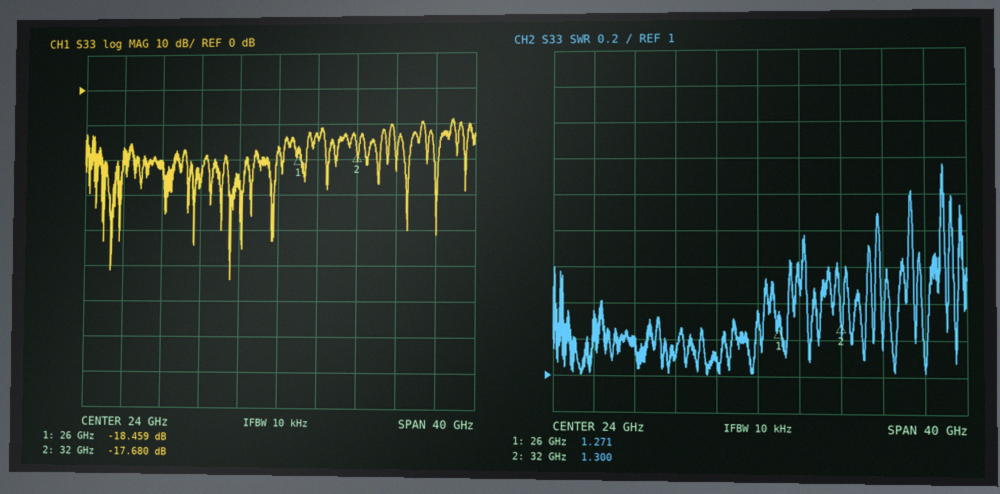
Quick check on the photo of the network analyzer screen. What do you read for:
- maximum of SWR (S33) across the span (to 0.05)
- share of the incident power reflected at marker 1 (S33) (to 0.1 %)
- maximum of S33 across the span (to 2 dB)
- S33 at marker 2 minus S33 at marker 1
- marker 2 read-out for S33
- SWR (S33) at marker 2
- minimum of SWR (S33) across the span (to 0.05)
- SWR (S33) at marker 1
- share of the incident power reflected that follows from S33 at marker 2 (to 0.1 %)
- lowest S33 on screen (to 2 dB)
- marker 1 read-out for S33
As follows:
2.15
1.4 %
-8 dB
0.779 dB
-17.680 dB
1.300
1.00
1.271
1.7 %
-54 dB
-18.459 dB
